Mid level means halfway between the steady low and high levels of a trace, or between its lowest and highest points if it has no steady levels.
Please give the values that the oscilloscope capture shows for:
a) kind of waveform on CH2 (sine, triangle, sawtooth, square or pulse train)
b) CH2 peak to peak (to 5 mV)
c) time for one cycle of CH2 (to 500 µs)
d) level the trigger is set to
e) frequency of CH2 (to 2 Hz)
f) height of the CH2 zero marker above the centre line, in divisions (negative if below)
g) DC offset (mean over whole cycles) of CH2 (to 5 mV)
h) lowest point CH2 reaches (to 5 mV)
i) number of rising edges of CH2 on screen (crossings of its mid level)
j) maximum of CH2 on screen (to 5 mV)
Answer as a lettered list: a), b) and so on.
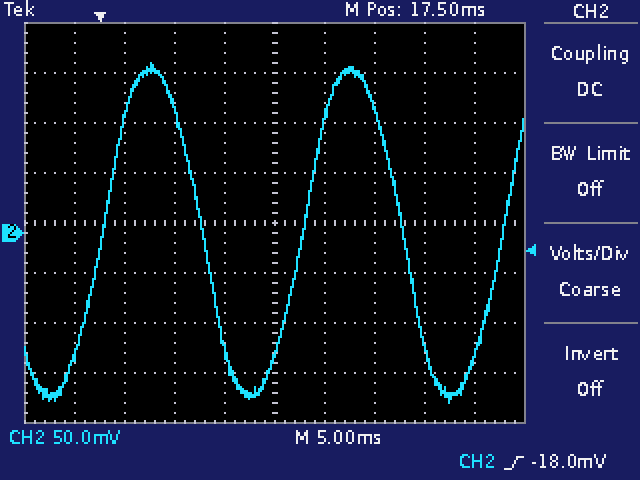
a) sine
b) 340 mV
c) 20.0 ms
d) -18.0 mV
e) 50 Hz
f) -0.2 div
g) 0 mV
h) -170 mV
i) 3
j) 170 mV
